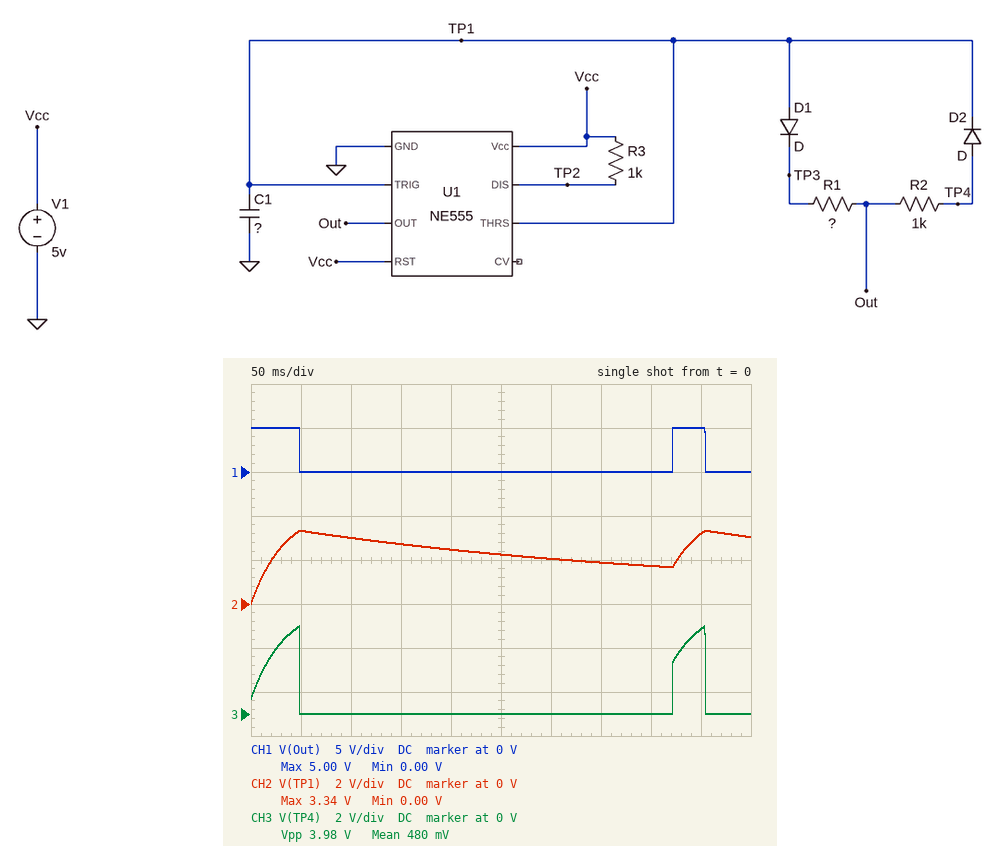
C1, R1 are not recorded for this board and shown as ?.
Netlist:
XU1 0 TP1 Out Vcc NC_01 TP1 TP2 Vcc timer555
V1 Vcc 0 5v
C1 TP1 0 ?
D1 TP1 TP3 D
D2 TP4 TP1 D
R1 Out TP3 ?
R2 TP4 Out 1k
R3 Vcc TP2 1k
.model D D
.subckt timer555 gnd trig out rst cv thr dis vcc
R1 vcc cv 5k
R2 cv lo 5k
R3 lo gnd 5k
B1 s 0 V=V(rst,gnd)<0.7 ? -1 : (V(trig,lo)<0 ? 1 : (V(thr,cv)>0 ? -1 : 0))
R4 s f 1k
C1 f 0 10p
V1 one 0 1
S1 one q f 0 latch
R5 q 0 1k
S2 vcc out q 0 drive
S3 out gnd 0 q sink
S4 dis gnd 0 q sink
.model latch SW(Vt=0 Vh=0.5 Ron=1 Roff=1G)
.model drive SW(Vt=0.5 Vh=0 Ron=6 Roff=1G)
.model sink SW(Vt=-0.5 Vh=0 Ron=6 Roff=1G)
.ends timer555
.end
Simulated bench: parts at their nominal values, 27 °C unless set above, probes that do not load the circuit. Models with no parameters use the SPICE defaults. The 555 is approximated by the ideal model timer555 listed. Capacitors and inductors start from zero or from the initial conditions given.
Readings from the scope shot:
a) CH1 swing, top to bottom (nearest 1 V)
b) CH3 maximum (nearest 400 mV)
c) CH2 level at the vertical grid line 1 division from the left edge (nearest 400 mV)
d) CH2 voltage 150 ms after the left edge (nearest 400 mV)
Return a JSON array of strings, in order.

["5 V", "4.0 V", "3.2 V", "2.8 V"]
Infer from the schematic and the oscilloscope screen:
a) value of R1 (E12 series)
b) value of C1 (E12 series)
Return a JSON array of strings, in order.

["12 kΩ", "33 µF"]
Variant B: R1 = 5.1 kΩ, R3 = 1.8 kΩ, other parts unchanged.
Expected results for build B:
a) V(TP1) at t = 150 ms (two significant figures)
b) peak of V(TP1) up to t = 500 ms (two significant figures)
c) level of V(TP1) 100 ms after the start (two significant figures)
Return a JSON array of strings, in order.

["2.1 V", "3.3 V", "2.6 V"]
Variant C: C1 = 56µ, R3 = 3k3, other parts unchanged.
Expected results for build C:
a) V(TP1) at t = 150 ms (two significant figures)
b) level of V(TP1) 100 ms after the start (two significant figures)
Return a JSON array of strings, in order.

["3.1 V", "3.3 V"]
